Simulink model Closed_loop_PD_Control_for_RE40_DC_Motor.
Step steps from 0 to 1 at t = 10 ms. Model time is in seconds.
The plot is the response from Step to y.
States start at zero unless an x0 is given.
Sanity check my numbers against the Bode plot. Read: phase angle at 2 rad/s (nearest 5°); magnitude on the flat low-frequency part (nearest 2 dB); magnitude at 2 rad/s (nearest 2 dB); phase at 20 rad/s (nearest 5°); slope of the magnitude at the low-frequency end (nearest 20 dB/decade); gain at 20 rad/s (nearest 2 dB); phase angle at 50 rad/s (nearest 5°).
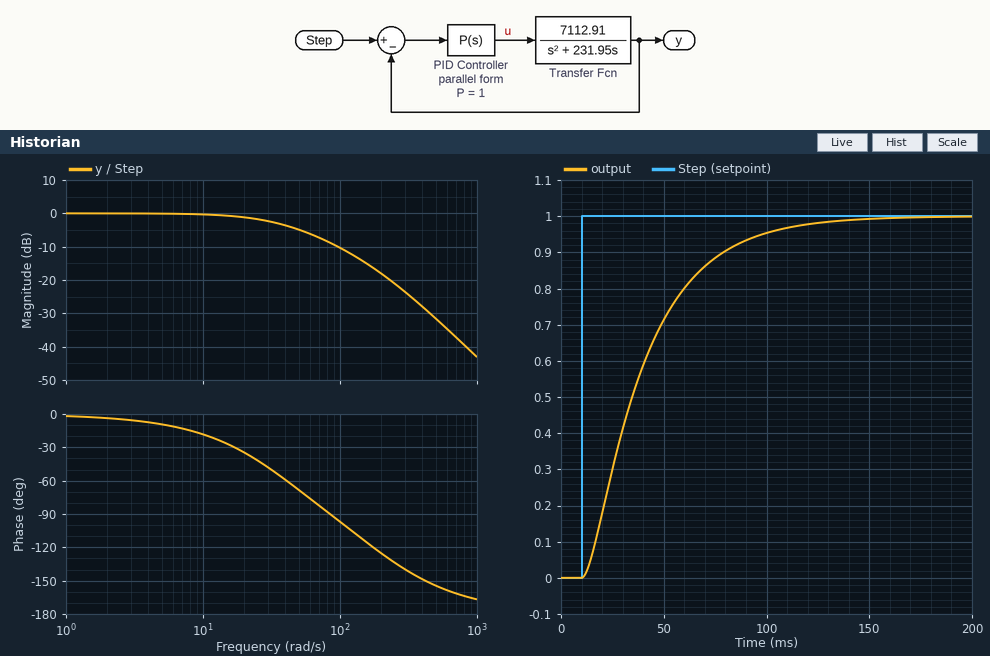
-5°
0 dB
0 dB
-35°
0 dB/decade
-2 dB
-70°
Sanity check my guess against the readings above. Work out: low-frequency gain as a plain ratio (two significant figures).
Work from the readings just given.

1.0
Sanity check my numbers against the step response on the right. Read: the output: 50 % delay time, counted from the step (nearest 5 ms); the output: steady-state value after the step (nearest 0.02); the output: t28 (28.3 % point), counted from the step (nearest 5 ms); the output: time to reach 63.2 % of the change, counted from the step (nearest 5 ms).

25 ms
1.00
15 ms
35 ms
